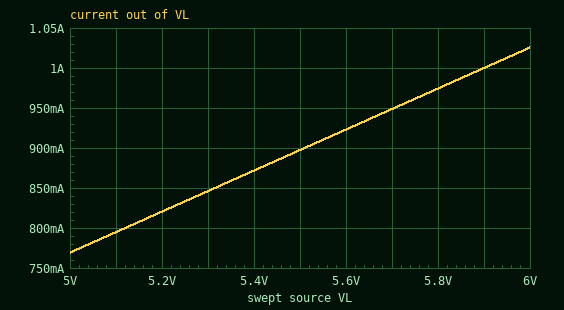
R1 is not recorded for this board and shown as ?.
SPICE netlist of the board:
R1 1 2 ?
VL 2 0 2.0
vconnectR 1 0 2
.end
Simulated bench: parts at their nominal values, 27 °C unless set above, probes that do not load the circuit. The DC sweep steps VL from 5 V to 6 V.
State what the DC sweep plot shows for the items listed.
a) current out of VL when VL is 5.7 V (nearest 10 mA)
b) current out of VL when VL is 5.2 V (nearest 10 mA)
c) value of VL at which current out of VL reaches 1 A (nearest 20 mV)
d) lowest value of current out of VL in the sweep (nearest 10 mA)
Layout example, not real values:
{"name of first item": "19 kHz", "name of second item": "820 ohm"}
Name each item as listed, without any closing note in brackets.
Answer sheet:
{"current out of VL when VL is 5.7 V": "950 mA", "current out of VL when VL is 5.2 V": "820 mA", "value of VL at which current out of VL reaches 1 A": "5.90 V", "lowest value of current out of VL in the sweep": "770 mA"}
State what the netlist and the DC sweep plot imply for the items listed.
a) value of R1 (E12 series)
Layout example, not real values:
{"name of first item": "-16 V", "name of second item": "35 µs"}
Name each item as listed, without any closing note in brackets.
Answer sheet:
{"value of R1": "3.9 Ω"}
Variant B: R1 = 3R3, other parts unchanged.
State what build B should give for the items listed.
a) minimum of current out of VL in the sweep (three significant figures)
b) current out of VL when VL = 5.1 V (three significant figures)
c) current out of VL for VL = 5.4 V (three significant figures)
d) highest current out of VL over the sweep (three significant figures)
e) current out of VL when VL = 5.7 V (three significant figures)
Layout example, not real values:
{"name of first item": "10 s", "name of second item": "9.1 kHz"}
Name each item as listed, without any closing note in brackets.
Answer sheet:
{"minimum of current out of VL in the sweep": "909 mA", "current out of VL when VL = 5.1 V": "939 mA", "current out of VL for VL = 5.4 V": "1.03 A", "highest current out of VL over the sweep": "1.21 A", "current out of VL when VL = 5.7 V": "1.12 A"}
